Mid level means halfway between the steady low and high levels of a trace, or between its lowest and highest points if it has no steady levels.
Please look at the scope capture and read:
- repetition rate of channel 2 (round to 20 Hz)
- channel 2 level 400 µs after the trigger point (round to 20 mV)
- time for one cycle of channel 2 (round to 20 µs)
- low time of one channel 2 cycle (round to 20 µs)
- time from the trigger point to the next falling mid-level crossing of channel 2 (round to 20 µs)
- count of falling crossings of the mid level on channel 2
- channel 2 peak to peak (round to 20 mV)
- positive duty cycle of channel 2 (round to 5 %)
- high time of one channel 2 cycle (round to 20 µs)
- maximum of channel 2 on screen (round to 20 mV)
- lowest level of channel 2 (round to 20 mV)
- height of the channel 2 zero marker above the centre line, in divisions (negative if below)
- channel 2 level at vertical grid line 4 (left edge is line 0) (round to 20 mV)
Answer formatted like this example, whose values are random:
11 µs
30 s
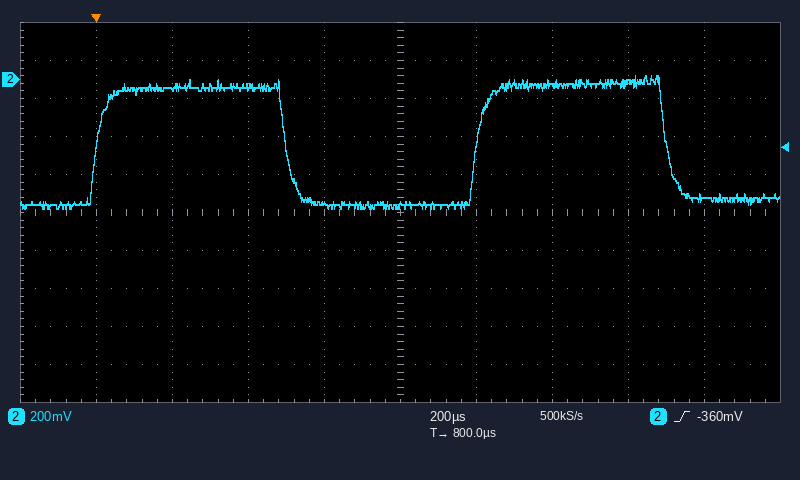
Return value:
1.00 kHz
-40 mV
1.00 ms
500 µs
500 µs
2
700 mV
50 %
500 µs
20 mV
-680 mV
+3.5 div
-660 mV
